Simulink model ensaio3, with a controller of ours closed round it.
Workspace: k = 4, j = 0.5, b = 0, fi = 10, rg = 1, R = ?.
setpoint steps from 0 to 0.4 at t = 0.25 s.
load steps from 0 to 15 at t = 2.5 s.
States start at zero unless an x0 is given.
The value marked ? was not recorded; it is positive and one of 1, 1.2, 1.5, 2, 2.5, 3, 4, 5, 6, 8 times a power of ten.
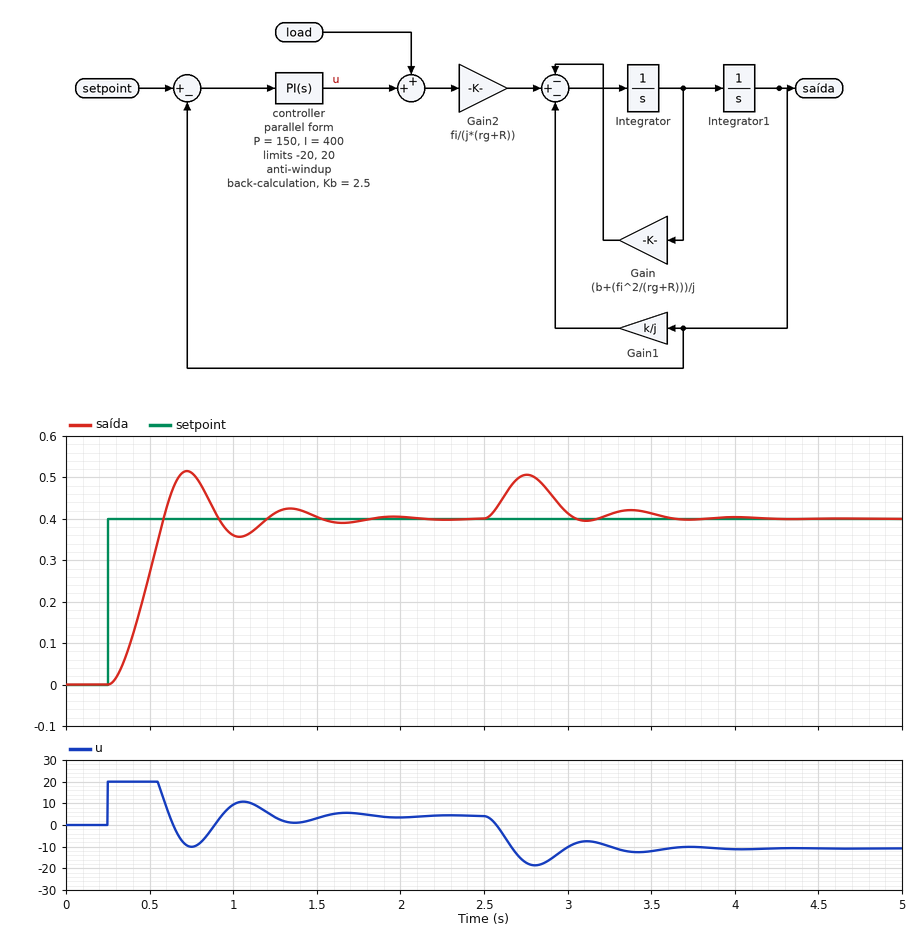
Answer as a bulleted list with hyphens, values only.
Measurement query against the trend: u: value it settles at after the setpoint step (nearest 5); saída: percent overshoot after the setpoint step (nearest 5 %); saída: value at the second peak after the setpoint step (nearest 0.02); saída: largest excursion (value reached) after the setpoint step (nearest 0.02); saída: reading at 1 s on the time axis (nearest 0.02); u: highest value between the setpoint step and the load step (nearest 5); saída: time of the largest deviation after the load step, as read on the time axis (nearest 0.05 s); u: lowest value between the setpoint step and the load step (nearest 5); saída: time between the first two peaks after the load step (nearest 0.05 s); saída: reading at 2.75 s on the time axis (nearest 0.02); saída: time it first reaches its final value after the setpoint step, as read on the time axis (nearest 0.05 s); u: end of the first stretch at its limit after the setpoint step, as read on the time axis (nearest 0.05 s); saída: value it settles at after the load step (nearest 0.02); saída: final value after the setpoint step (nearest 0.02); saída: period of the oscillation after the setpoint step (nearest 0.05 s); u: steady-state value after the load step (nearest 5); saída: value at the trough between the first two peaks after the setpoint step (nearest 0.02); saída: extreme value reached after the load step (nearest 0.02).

- 5
- 30 %
- 0.42
- 0.52
- 0.36
- 20
- 2.75 s
- -10
- 0.60 s
- 0.50
- 0.60 s
- 0.55 s
- 0.40
- 0.40
- 0.60 s
- -10
- 0.36
- 0.50
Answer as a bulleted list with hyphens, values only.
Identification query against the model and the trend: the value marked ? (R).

- 25
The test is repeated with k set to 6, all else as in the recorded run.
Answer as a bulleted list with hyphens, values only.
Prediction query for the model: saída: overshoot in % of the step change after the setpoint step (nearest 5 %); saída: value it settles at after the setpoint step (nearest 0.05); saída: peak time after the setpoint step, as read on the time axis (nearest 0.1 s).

- 25 %
- 0.40
- 0.7 s
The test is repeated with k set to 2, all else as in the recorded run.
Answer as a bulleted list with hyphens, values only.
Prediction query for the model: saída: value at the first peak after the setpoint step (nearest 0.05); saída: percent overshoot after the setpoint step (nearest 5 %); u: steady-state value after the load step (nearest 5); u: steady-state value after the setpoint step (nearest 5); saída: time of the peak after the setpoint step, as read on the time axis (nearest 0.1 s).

- 0.55
- 35 %
- -15
- 0
- 0.7 s
